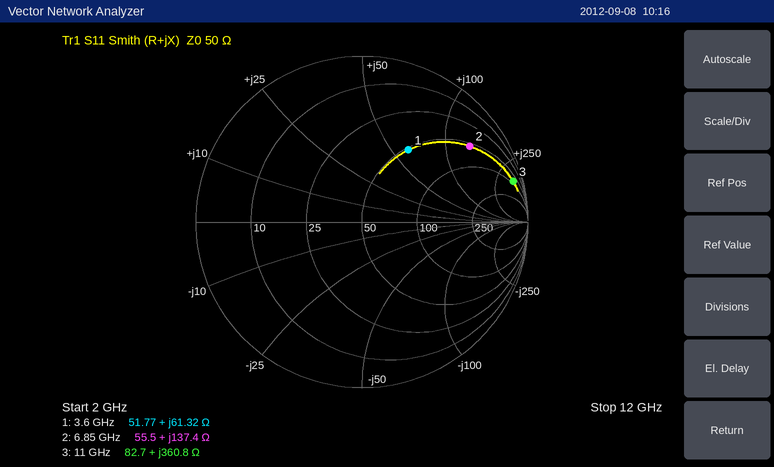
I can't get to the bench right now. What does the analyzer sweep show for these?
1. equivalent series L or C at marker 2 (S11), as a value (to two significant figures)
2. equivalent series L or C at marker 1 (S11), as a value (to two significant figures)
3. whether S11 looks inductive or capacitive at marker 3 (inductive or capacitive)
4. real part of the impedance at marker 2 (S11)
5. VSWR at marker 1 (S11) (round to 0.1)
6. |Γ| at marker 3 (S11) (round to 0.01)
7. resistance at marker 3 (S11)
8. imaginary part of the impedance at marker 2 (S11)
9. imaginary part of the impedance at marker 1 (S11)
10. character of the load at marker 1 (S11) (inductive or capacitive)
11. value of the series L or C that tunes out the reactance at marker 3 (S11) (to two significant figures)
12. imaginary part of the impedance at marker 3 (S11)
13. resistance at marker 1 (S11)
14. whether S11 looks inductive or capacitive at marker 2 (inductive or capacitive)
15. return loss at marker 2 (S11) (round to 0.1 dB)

3.2 nH
2.7 nH
inductive
55.5 Ω
3.1
0.94
82.7 Ω
+137.4 Ω
+61.32 Ω
inductive
40 fF
+360.8 Ω
51.77 Ω
inductive
2.0 dB
